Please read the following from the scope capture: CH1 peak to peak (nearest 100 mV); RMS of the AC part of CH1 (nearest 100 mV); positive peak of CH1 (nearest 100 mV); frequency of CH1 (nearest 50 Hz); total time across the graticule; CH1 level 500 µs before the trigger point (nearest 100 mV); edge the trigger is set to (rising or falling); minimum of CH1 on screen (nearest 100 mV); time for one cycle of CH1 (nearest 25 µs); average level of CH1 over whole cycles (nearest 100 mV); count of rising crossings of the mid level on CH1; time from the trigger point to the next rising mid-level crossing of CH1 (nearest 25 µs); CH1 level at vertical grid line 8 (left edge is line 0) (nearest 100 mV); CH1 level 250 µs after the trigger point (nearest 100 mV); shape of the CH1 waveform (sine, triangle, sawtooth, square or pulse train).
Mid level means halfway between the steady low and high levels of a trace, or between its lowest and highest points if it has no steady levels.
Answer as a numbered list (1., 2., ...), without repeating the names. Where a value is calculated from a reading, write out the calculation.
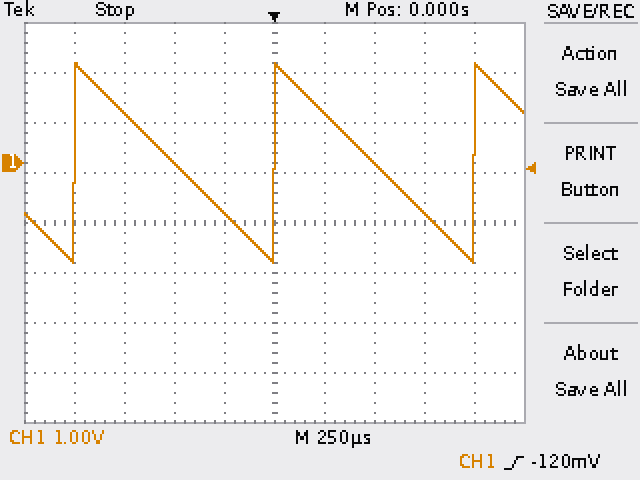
1. 2.0 V − (-2.0 V) = 4.0 V
2. 4.0 V / (2√3) ≈ 1.2 V
3. 2.0 V
4. 1 / 1.000 ms ≈ 1.00 kHz
5. 2.5 ms
6. 0.0 V
7. rising
8. -2.0 V
9. 1.000 ms
10. (2.0 V + (-2.0 V)) / 2 ≈ 0.0 V
11. 3
12. 1.000 ms
13. -1.0 V
14. 1.0 V
15. sawtooth
